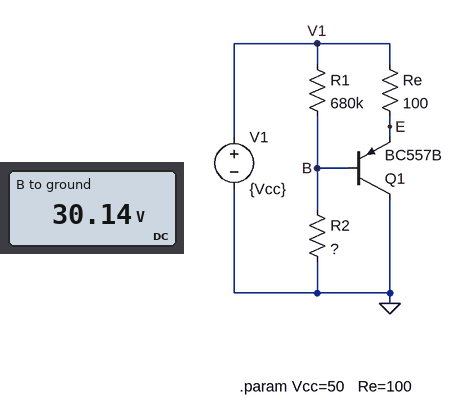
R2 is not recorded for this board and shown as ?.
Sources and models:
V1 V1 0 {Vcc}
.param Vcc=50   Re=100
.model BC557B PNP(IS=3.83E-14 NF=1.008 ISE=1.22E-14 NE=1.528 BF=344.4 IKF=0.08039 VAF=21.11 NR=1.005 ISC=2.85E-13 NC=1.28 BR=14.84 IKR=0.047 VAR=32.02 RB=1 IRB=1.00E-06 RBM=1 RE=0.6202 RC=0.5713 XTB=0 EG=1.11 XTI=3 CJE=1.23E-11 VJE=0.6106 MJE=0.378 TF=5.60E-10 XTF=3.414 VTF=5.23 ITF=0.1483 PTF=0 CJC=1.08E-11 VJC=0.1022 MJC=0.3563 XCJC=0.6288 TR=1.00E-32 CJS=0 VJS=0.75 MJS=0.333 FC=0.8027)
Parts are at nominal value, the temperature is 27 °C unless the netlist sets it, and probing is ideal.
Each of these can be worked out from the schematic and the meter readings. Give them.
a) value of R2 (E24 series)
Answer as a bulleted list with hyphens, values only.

- 62 kΩ
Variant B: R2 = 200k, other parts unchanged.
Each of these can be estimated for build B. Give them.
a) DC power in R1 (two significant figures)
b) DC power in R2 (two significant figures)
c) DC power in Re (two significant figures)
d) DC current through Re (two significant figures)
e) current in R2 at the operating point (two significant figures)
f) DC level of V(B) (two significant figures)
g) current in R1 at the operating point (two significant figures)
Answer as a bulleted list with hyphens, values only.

- 210 µW
- 7.3 mW
- 1.2 W
- 110 mA
- 190 µA
- 38 V
- 17 µA
